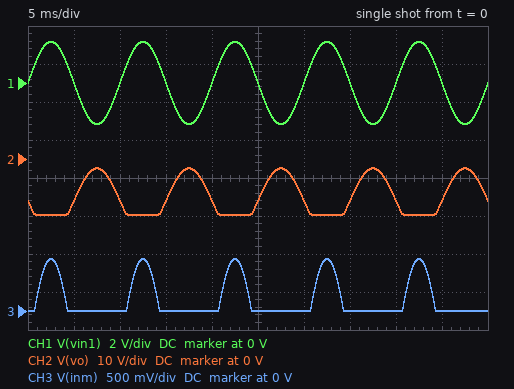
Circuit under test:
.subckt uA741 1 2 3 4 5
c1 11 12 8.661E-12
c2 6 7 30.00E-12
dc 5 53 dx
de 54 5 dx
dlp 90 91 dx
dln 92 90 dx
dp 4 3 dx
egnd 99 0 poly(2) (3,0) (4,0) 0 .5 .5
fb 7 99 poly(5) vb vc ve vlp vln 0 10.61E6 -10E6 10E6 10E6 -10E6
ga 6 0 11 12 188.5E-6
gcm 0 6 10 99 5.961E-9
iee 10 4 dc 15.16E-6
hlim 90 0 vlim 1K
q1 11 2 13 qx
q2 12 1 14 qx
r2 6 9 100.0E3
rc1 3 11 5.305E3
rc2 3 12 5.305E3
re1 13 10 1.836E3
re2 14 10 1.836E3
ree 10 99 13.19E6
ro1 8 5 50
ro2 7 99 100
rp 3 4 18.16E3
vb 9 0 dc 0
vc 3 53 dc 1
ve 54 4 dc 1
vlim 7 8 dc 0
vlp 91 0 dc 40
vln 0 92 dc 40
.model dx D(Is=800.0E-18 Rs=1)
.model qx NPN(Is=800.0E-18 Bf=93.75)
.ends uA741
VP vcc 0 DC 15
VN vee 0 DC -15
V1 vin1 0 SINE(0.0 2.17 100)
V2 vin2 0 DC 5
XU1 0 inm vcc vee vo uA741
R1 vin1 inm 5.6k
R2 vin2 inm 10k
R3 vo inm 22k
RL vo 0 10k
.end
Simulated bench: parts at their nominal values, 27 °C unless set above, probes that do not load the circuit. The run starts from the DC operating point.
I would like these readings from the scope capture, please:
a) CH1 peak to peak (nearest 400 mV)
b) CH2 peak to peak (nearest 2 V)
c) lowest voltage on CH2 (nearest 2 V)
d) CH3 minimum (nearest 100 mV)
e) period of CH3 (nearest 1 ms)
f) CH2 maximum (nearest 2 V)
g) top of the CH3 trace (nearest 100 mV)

4.4 V
12 V
-14 V
0 V
10 ms
-2 V
700 mV
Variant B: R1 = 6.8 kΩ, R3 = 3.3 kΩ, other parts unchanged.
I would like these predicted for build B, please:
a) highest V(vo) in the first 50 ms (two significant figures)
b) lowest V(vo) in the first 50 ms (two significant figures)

-600 mV
-2.7 V
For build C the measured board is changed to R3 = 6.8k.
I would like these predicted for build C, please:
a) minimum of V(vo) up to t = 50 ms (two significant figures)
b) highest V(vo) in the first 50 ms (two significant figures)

-6.0 V
-760 mV
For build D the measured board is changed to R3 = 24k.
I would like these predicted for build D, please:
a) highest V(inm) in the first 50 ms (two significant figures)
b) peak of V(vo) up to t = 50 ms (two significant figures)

870 mV
-2.7 V
